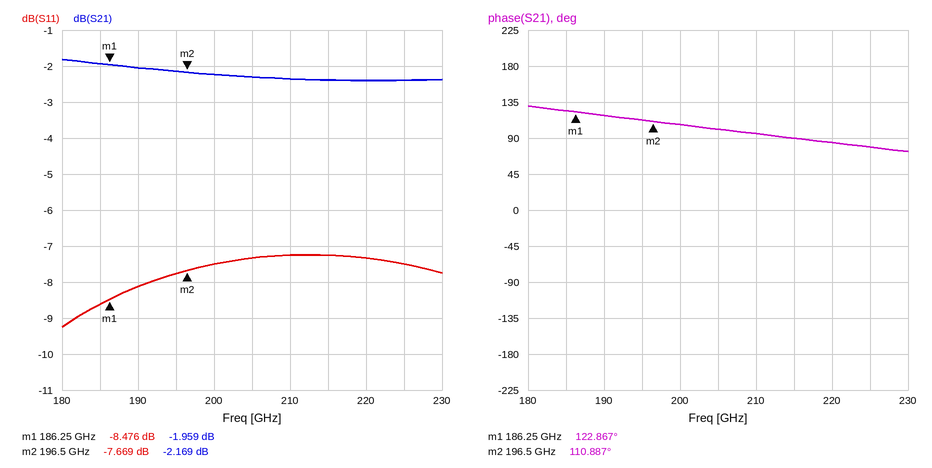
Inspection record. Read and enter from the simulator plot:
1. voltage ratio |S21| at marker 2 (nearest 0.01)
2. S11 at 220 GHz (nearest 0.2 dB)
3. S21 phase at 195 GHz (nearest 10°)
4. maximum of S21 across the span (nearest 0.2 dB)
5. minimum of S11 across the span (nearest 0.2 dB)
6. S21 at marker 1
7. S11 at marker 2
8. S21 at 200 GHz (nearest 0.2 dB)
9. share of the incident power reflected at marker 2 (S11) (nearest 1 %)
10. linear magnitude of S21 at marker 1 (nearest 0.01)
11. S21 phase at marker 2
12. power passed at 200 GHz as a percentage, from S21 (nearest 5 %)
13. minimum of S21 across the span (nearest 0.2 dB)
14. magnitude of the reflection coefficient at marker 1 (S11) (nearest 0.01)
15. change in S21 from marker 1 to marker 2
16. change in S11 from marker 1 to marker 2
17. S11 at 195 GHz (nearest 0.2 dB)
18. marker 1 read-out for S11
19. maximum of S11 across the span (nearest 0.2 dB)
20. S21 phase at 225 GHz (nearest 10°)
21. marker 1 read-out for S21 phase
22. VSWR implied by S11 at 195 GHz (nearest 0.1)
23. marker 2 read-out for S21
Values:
0.78
-7.4 dB
110°
-1.8 dB
-9.2 dB
-1.959 dB
-7.669 dB
-2.2 dB
17 %
0.80
110.887°
60 %
-2.4 dB
0.38
-0.210 dB
0.807 dB
-7.8 dB
-8.476 dB
-7.2 dB
80°
122.867°
2.4
-2.169 dB
